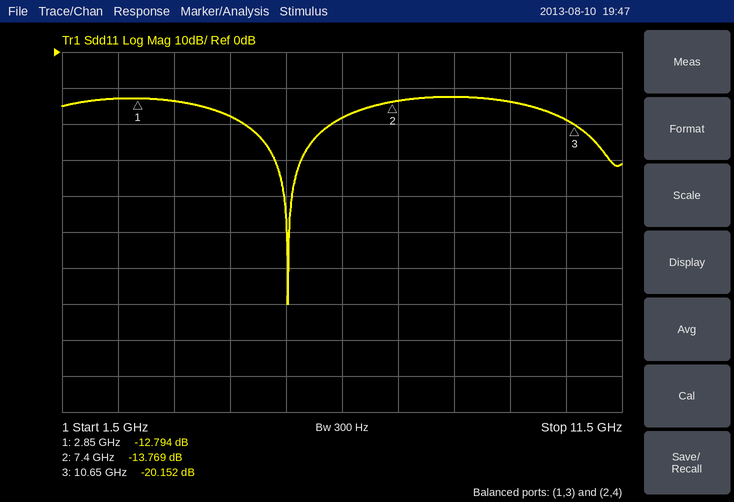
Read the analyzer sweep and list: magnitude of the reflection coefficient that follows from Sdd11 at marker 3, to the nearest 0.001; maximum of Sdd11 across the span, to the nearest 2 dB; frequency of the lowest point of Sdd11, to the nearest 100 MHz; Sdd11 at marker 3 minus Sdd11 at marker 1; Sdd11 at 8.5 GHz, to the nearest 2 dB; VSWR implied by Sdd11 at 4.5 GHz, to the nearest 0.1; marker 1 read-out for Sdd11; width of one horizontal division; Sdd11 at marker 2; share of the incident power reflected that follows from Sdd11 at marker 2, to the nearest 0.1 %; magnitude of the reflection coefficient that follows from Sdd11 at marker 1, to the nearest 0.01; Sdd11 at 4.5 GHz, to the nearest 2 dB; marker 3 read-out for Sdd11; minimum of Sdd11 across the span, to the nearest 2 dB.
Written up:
0.098
-12 dB
5.5 GHz
-7.358 dB
-12 dB
1.3
-12.794 dB
1 GHz
-13.769 dB
4.2 %
0.23
-18 dB
-20.152 dB
-70 dB
